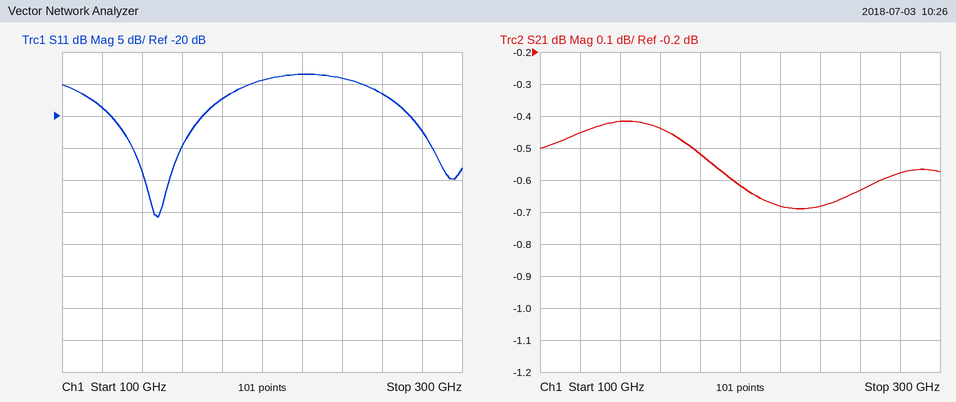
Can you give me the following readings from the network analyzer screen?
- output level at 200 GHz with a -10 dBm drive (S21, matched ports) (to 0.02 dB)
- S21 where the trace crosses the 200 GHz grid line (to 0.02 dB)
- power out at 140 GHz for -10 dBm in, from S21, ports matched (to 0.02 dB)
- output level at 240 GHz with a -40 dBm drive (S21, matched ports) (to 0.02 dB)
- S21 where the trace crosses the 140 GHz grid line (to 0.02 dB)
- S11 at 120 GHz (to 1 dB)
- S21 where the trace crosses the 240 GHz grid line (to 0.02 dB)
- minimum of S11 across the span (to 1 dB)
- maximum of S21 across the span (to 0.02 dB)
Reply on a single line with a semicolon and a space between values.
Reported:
-10.62 dBm; -0.62 dB; -10.42 dBm; -40.68 dBm; -0.42 dB; -19 dB; -0.68 dB; -36 dB; -0.42 dB
